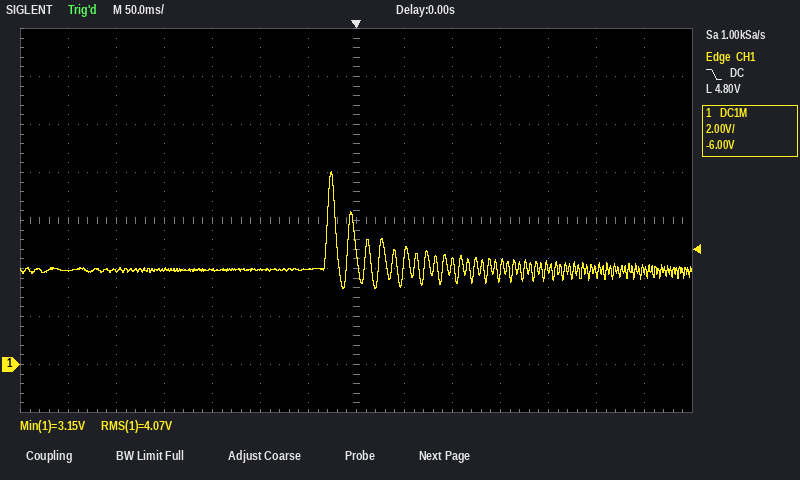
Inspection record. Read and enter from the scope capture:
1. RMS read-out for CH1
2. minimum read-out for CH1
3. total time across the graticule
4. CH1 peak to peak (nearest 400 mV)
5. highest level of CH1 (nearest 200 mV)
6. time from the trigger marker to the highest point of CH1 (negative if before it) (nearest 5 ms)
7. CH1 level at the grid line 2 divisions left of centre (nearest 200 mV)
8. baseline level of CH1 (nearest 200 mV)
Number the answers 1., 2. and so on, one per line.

1. 4.07 V
2. 3.15 V
3. 700 ms
4. 4.8 V
5. 8.0 V
6. -25 ms
7. 4.0 V
8. 4.0 V
